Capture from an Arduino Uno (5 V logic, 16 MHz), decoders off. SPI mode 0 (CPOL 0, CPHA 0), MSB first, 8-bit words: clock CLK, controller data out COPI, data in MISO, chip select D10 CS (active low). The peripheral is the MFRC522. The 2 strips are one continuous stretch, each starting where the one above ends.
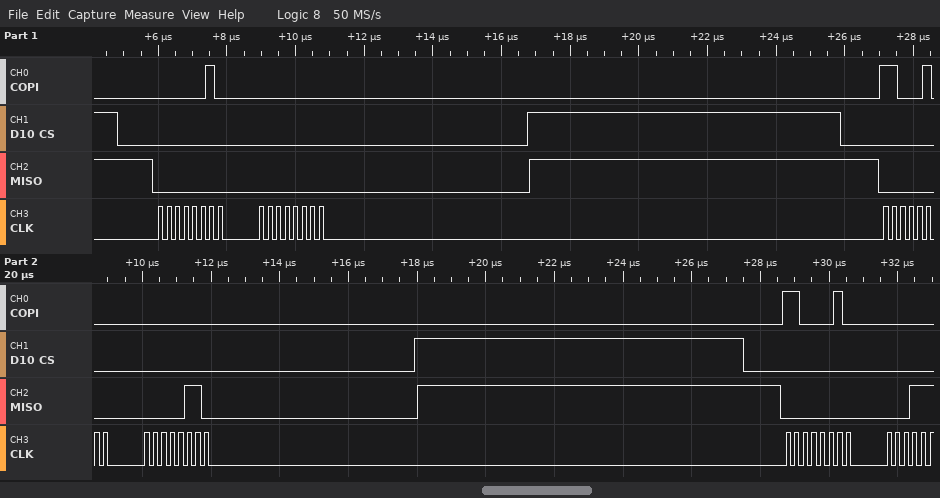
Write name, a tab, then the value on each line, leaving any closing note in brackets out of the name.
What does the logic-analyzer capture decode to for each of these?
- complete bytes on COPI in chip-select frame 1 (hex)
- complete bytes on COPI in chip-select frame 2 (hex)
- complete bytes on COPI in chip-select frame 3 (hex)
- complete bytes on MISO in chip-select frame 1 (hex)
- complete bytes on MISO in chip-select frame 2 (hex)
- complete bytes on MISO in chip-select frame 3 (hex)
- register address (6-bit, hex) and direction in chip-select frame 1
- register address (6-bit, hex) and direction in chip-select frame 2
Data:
complete bytes on COPI in chip-select frame 1	02 00
complete bytes on COPI in chip-select frame 2	C4 00
complete bytes on COPI in chip-select frame 3	C2
complete bytes on MISO in chip-select frame 1	00 00
complete bytes on MISO in chip-select frame 2	00 06
complete bytes on MISO in chip-select frame 3	00
register address (6-bit, hex) and direction in chip-select frame 1	0x01 write
register address (6-bit, hex) and direction in chip-select frame 2	0x22 read
